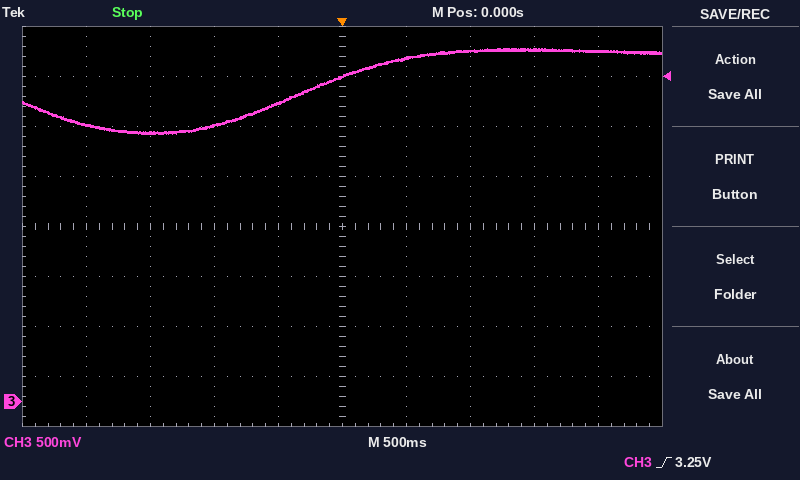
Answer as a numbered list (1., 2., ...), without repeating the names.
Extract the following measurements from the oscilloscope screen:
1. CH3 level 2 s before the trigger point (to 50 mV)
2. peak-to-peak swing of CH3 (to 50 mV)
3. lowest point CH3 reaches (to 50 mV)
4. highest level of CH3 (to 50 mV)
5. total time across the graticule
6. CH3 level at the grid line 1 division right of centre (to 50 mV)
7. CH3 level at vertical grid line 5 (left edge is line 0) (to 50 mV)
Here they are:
1. 2.75 V
2. 850 mV
3. 2.70 V
4. 3.55 V
5. 5 s
6. 3.45 V
7. 3.25 V
